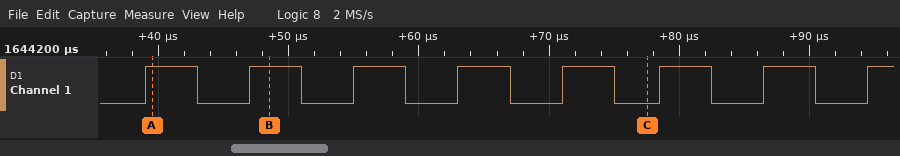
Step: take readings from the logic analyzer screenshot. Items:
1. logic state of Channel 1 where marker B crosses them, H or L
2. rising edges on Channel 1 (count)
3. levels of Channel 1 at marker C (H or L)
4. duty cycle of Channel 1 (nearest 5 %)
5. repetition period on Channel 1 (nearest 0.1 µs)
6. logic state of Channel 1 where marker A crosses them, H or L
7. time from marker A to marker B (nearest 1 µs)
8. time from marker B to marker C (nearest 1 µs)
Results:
Channel 1=H
8
Channel 1=L
50 %
7.9 µs
Channel 1=H
9 µs
29 µs
